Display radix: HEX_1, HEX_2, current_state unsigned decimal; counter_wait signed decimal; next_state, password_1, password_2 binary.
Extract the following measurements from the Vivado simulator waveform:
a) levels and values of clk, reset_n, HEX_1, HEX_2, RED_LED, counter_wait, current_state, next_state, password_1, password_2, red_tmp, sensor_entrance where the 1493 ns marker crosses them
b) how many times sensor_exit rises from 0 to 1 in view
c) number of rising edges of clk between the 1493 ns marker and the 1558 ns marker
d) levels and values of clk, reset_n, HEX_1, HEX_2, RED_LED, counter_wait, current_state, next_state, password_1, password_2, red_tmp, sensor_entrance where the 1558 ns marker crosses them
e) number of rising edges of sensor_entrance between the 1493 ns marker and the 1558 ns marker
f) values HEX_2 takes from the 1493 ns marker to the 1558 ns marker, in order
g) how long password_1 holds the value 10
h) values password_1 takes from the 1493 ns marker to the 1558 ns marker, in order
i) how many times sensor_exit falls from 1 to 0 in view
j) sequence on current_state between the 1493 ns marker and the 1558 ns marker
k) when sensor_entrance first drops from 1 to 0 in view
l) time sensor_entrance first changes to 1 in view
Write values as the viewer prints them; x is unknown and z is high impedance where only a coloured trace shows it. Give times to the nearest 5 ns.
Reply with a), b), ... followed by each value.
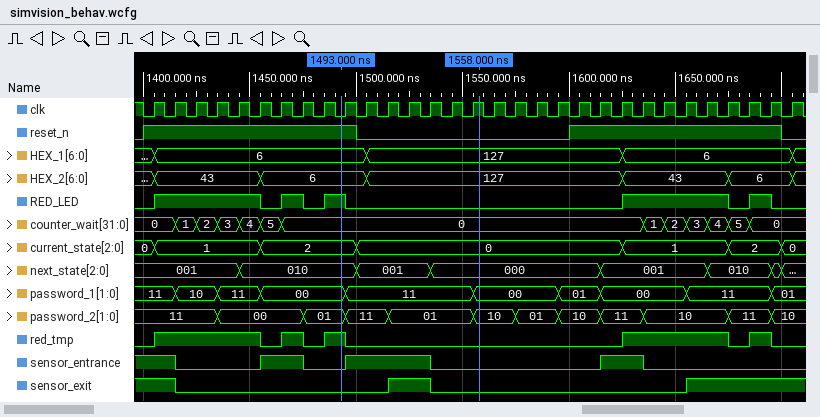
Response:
a) clk=0, reset_n=1, HEX_1=6, HEX_2=6, RED_LED=1, counter_wait=0, current_state=2, next_state=010, password_1=00, password_2=01, red_tmp=1, sensor_entrance=0
b) 2
c) 7
d) clk=1, reset_n=0, HEX_1=127, HEX_2=127, RED_LED=0, counter_wait=0, current_state=0, next_state=000, password_1=00, password_2=10, red_tmp=0, sensor_entrance=0
e) 1
f) 6, 127
g) 20 ns
h) 00, 11, 00
i) 2
j) 2, 0
k) 1415 ns
l) 1455 ns
